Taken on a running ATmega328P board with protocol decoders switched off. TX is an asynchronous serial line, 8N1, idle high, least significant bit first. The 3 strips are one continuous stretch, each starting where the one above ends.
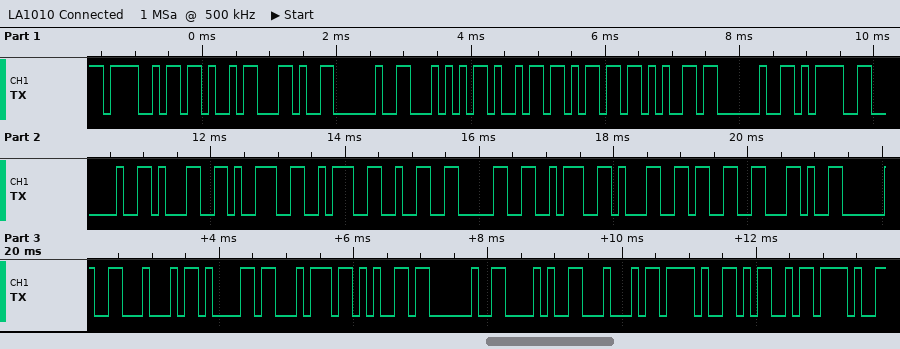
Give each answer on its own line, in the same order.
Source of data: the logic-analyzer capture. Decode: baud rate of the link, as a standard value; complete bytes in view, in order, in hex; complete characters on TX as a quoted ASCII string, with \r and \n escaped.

9600 baud
4F 4B 2C 20 54 69 6D 65 20 3D 20 31 39 3A 32 30 3A 31 33 2C 20 44 61 74 65 20 28 44 2F 4D 2F
"OK, Time = 19:20:13, Date (D/M/"
